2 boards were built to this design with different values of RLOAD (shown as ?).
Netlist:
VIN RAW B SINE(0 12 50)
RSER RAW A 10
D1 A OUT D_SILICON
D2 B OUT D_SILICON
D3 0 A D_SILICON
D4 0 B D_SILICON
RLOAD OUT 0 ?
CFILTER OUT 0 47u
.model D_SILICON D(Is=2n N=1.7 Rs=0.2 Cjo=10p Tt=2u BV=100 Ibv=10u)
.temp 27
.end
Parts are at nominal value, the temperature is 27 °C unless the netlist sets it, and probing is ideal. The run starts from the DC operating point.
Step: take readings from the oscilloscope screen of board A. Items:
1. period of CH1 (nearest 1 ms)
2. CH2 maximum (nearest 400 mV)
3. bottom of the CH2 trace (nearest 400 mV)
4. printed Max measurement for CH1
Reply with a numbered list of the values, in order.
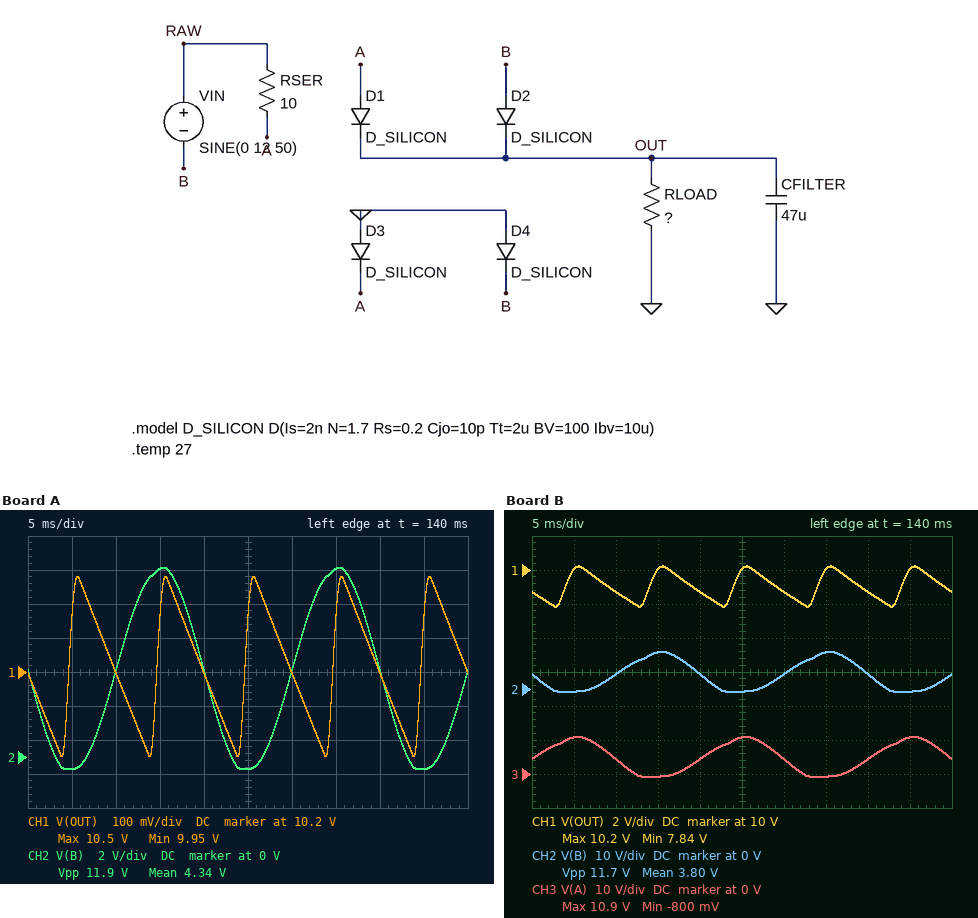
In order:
1. 10 ms
2. 11.2 V
3. -800 mV
4. 10.5 V
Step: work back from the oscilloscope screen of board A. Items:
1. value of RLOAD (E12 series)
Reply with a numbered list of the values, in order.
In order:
1. 3.3 kΩ
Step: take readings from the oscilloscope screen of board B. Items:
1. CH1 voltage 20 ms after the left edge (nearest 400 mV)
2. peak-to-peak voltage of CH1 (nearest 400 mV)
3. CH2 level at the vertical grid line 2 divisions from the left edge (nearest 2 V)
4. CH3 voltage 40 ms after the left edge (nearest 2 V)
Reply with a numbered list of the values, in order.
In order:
1. 8.8 V
2. 2.4 V
3. 4 V
4. 4 V
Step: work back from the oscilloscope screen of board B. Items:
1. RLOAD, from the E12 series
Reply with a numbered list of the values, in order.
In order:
1. 560 Ω
